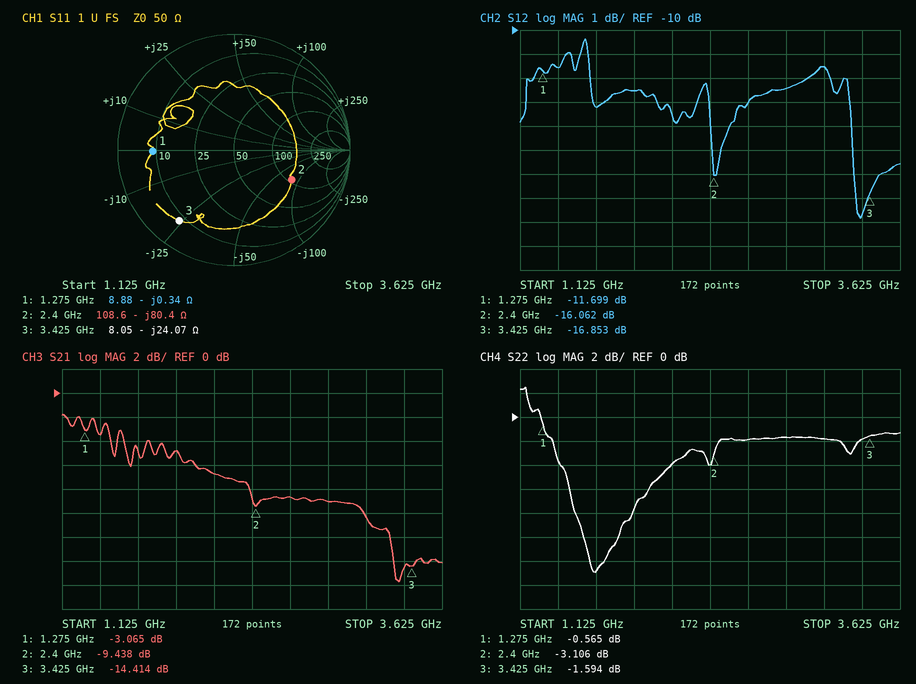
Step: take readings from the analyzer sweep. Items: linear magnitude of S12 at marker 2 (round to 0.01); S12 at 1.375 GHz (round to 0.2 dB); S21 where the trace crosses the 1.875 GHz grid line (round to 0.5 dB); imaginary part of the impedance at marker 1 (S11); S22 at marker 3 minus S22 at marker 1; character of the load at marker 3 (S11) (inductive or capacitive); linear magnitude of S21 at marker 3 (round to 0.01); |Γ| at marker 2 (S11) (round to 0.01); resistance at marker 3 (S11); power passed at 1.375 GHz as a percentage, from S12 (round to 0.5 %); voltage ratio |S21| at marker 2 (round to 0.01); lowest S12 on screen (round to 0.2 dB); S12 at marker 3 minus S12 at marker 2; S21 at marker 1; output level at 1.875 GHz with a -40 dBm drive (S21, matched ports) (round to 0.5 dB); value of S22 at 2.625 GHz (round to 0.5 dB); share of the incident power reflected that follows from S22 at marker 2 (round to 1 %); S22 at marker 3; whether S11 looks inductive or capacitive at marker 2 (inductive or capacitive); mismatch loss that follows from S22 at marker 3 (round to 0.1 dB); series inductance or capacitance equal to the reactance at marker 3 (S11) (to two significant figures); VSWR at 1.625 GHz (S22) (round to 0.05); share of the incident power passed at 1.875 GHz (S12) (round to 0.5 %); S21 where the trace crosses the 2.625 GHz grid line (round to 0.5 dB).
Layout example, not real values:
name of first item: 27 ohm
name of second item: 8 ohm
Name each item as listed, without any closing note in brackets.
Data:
linear magnitude of S12 at marker 2: 0.16
S12 at 1.375 GHz: -11.6 dB
S21 where the trace crosses the 1.875 GHz grid line: -5.0 dB
imaginary part of the impedance at marker 1: -0.34 Ω
S22 at marker 3 minus S22 at marker 1: -1.029 dB
character of the load at marker 3 (S11): capacitive
linear magnitude of S21 at marker 3: 0.19
|Γ| at marker 2 (S11): 0.56
resistance at marker 3: 8.05 Ω
power passed at 1.375 GHz as a percentage, from S12: 7.0 %
voltage ratio |S21| at marker 2: 0.34
lowest S12 on screen: -17.8 dB
S12 at marker 3 minus S12 at marker 2: -0.791 dB
S21 at marker 1: -3.065 dB
output level at 1.875 GHz with a -40 dBm drive (S21, matched ports): -45.0 dBm
value of S22 at 2.625 GHz: -2.0 dB
share of the incident power reflected that follows from S22 at marker 2: 49 %
S22 at marker 3: -1.594 dB
whether S11 looks inductive or capacitive at marker 2: capacitive
mismatch loss that follows from S22 at marker 3: 5.1 dB
series inductance or capacitance equal to the reactance at marker 3 (S11): 1.9 pF
VSWR at 1.625 GHz (S22): 1.60
share of the incident power passed at 1.875 GHz (S12): 5.5 %
S21 where the trace crosses the 2.625 GHz grid line: -8.5 dB
